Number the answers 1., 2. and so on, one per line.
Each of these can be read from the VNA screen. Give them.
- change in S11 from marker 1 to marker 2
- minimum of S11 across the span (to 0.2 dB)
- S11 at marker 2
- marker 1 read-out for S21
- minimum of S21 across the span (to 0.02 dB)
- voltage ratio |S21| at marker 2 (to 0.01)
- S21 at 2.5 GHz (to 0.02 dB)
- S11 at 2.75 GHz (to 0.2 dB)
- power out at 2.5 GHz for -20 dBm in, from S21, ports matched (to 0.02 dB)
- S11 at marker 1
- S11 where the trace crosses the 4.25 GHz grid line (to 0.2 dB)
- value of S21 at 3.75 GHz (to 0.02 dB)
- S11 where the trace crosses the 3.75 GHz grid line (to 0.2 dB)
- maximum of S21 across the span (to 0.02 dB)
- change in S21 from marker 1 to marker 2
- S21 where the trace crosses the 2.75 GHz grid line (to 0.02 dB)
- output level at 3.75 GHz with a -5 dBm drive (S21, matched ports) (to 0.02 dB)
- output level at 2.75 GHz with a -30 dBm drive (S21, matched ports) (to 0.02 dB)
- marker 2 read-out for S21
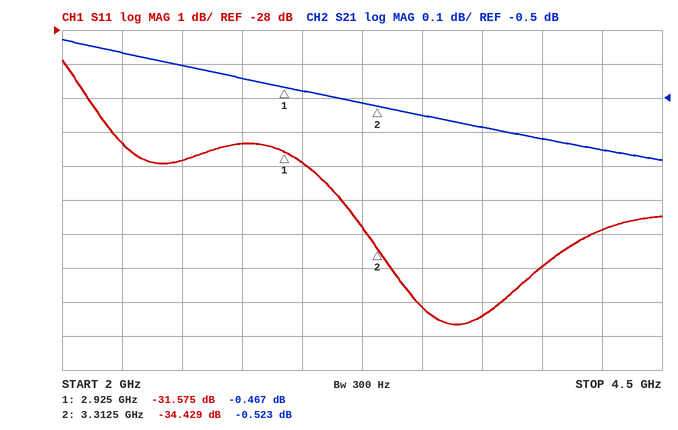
1. -2.854 dB
2. -36.6 dB
3. -34.429 dB
4. -0.467 dB
5. -0.68 dB
6. 0.94
7. -0.40 dB
8. -31.4 dB
9. -20.40 dBm
10. -31.575 dB
11. -33.8 dB
12. -0.58 dB
13. -36.4 dB
14. -0.32 dB
15. -0.056 dB
16. -0.44 dB
17. -5.58 dBm
18. -30.44 dBm
19. -0.523 dB
